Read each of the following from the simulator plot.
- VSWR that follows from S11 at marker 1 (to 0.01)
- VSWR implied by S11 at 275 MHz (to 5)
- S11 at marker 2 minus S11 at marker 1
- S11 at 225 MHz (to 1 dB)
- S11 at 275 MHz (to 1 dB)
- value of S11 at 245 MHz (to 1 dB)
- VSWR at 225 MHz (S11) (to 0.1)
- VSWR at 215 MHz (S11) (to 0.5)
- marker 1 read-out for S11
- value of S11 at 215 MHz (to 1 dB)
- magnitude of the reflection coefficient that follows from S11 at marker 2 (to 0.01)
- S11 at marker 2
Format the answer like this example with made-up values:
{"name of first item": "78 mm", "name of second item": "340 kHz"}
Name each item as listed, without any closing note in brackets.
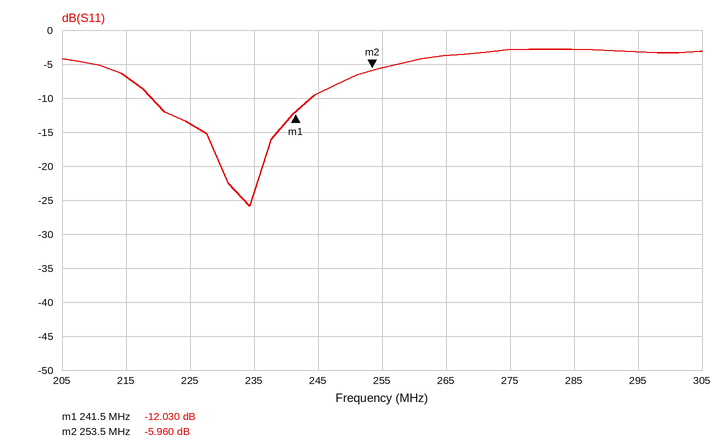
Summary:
{"VSWR that follows from S11 at marker 1": "1.67", "VSWR implied by S11 at 275 MHz": "5", "S11 at marker 2 minus S11 at marker 1": "6.070 dB", "S11 at 225 MHz": "-14 dB", "S11 at 275 MHz": "-3 dB", "value of S11 at 245 MHz": "-9 dB", "VSWR at 225 MHz (S11)": "1.5", "VSWR at 215 MHz (S11)": "2.5", "marker 1 read-out for S11": "-12.030 dB", "value of S11 at 215 MHz": "-7 dB", "magnitude of the reflection coefficient that follows from S11 at marker 2": "0.50", "S11 at marker 2": "-5.960 dB"}
